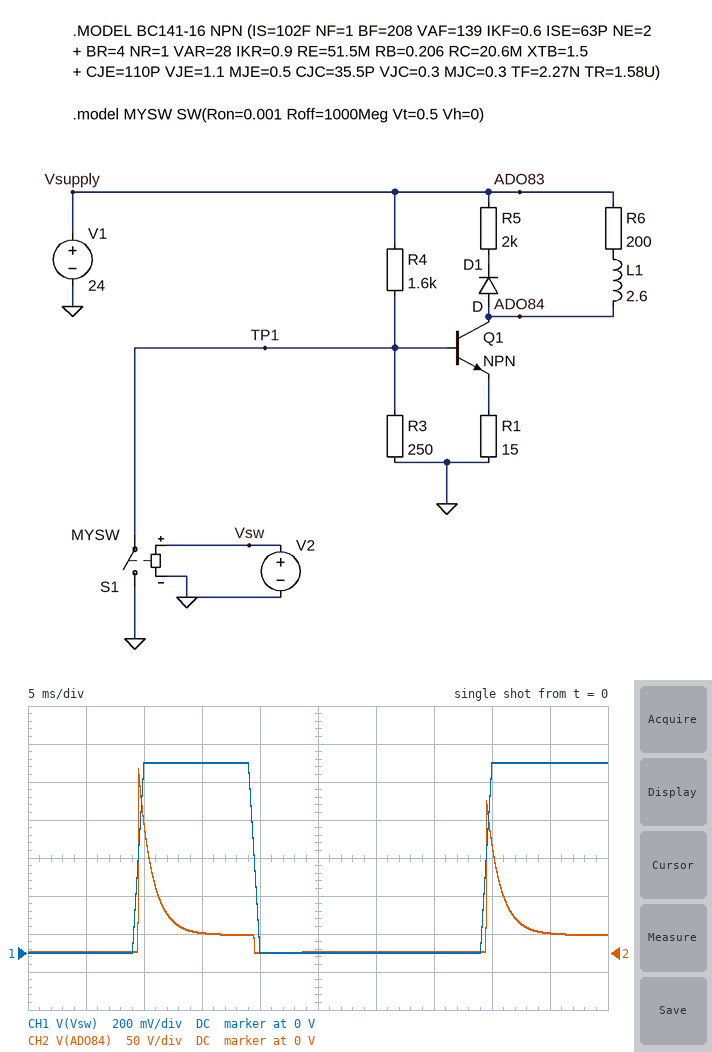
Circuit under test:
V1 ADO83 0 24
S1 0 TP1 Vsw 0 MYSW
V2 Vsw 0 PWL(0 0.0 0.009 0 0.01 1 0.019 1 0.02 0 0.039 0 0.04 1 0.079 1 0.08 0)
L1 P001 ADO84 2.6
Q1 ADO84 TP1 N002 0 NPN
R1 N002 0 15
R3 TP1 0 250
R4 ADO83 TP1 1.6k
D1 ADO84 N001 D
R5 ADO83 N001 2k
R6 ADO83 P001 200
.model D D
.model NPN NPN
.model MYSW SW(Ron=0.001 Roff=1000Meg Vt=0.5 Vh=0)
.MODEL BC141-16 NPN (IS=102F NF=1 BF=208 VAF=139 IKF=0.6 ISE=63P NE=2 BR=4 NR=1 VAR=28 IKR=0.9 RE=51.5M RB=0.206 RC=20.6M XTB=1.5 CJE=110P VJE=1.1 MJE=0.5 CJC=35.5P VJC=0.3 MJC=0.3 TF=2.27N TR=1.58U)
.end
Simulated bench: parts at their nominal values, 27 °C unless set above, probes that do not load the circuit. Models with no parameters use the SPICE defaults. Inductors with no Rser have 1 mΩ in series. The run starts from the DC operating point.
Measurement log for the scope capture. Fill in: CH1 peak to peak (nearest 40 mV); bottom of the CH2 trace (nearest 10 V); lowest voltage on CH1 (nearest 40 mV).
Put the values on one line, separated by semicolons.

1.00 V; 0 V; 0 V
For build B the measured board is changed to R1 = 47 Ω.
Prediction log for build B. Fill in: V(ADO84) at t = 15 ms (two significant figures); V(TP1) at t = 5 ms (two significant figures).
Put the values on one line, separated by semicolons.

25 V; 3.1 V
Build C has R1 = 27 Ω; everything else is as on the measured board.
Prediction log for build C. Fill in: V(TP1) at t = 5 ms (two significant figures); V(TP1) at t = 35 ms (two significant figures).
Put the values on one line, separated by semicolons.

3.1 V; 3.0 V
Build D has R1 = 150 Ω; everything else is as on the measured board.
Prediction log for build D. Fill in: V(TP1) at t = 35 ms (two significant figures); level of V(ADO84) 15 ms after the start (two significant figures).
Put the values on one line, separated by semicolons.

3.2 V; 24 V
